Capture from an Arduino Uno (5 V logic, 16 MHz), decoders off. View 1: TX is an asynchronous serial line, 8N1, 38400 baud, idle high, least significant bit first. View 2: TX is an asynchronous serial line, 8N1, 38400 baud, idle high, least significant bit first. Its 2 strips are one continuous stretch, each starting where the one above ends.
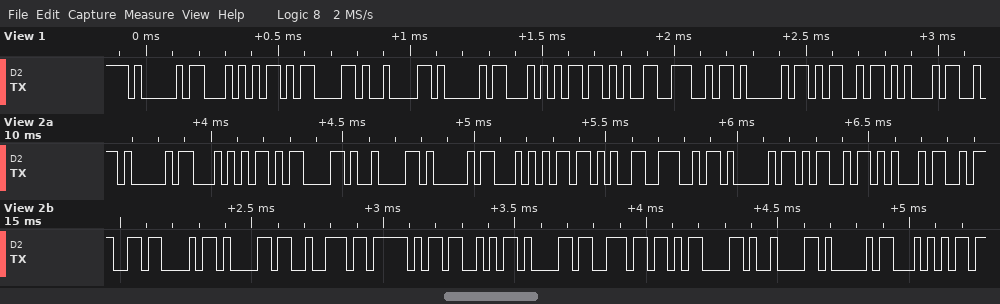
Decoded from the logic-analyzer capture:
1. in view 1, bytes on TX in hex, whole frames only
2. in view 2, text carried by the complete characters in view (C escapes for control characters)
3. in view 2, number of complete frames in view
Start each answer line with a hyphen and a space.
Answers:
- 0x41 0x54 0x0D 0x09 0x41 0x54 0x2B 0x4E 0x41 0x4D 0x45
- "AT\r\tAT+NAME:Car_San\r\tAT"
- 23
